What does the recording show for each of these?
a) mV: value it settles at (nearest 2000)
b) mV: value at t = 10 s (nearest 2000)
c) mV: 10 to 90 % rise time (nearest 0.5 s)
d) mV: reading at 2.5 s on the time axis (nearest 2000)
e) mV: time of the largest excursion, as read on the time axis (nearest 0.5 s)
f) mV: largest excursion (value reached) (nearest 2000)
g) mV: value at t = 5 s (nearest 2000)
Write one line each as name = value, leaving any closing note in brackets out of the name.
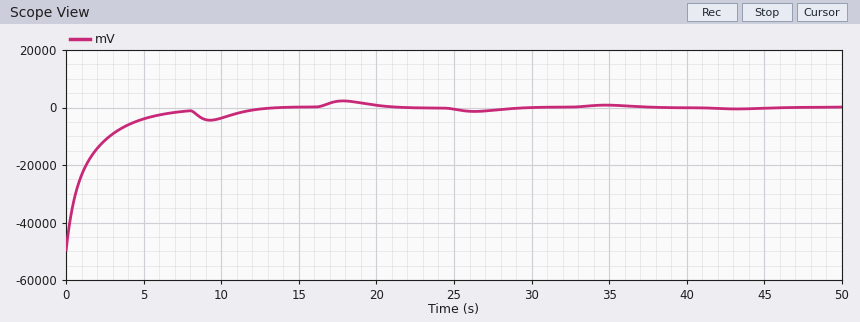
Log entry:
mV: value it settles at = 0
mV: value at t = 10 s = -4000
mV: 10 to 90 % rise time = 4.5 s
mV: reading at 2.5 s on the time axis = -12000
mV: time of the largest excursion, as read on the time axis = 18.0 s
mV: largest excursion (value reached) = 2000
mV: value at t = 5 s = -4000
